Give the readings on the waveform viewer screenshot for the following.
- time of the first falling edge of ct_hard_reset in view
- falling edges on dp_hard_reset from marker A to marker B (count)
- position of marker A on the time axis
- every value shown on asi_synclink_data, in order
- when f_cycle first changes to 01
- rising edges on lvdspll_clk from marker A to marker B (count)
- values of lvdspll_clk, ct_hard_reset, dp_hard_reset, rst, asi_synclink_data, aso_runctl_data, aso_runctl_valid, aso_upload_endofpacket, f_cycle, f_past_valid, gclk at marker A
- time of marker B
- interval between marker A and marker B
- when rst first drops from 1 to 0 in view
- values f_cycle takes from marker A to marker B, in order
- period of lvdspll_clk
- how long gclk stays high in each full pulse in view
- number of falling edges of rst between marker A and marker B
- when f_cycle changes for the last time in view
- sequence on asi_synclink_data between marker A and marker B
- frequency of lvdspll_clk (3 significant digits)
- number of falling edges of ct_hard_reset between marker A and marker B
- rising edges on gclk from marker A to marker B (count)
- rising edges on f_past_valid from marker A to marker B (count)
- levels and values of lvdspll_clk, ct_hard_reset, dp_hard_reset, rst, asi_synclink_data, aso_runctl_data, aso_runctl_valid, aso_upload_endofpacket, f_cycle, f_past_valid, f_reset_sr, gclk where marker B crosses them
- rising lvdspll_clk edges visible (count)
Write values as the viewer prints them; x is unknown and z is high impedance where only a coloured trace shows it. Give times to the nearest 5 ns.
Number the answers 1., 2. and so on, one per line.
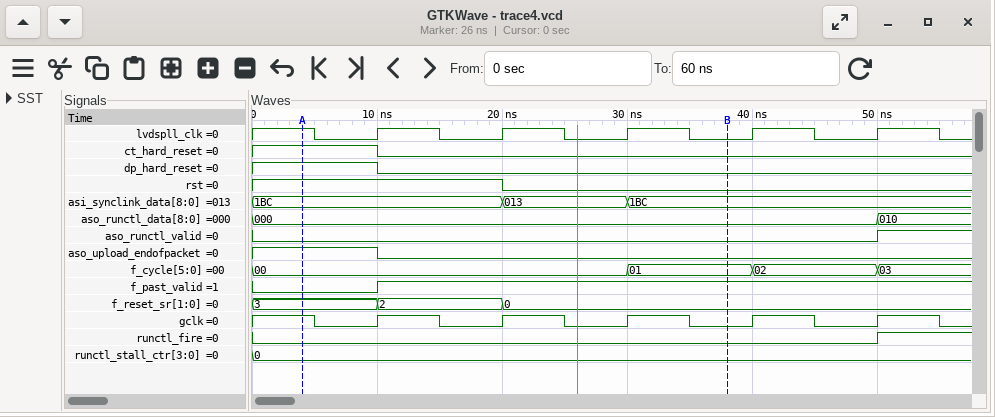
1. 10 ns
2. 1
3. 5 ns
4. 1BC, 013, 1BC
5. 30 ns
6. 3
7. lvdspll_clk=1, ct_hard_reset=1, dp_hard_reset=1, rst=1, asi_synclink_data=1BC, aso_runctl_data=000, aso_runctl_valid=0, aso_upload_endofpacket=1, f_cycle=00, f_past_valid=0, gclk=1
8. 40 ns
9. 35 ns
10. 20 ns
11. 00, 01
12. 10 ns
13. 5 ns, 5 ns, 5 ns, 5 ns, 5 ns
14. 1
15. 50 ns
16. 1BC, 013, 1BC
17. 100 MHz
18. 1
19. 3
20. 1
21. lvdspll_clk=0, ct_hard_reset=0, dp_hard_reset=0, rst=0, asi_synclink_data=1BC, aso_runctl_data=000, aso_runctl_valid=0, aso_upload_endofpacket=0, f_cycle=01, f_past_valid=1, f_reset_sr=0, gclk=0
22. 5
